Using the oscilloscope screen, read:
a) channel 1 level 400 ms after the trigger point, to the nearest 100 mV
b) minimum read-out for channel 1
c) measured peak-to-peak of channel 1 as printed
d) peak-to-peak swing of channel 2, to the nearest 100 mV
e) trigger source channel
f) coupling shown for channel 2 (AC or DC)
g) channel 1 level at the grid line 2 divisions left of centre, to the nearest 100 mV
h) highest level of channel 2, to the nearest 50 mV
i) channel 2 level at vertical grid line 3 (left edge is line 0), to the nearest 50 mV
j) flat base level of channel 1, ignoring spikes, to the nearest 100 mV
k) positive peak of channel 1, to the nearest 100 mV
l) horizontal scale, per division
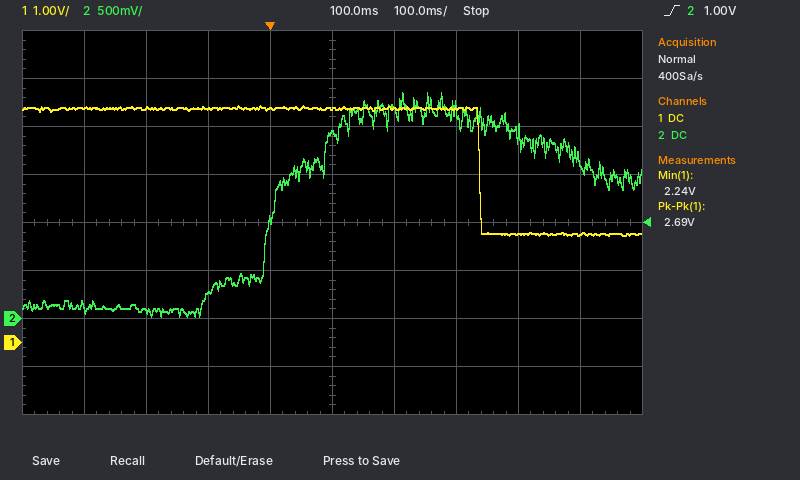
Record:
2.3 V
2.24 V
2.69 V
2.30 V
channel 2
DC
4.9 V
2.35 V
250 mV
2.3 V
4.9 V
100 ms
